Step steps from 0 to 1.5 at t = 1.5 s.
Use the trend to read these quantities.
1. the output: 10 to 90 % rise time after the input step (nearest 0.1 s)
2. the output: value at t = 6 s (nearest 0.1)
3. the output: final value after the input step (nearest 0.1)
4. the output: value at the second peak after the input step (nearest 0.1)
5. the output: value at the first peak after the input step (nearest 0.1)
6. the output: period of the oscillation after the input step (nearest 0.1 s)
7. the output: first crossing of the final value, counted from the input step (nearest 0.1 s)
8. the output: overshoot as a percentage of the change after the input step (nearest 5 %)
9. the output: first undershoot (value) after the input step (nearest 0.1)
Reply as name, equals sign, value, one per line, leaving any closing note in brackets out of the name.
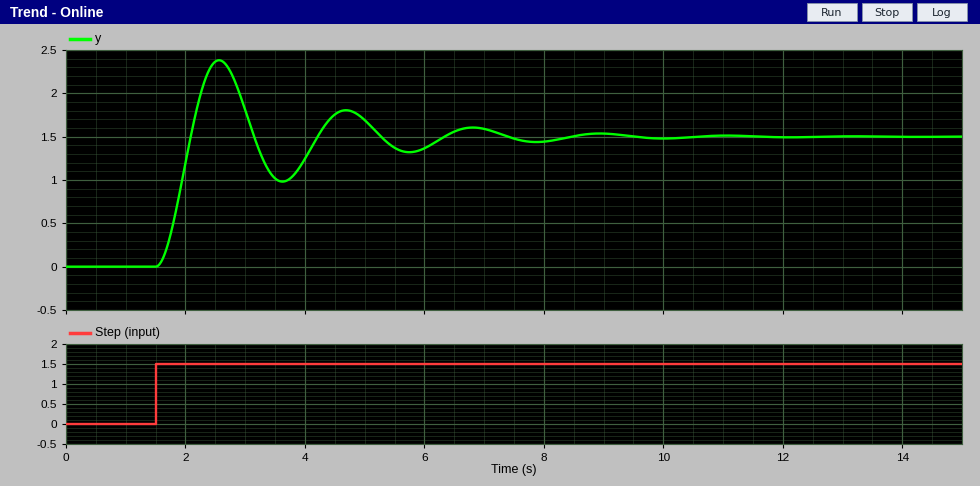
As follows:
the output: 10 to 90 % rise time after the input step = 0.4 s
the output: value at t = 6 s = 1.4
the output: final value after the input step = 1.5
the output: value at the second peak after the input step = 1.8
the output: value at the first peak after the input step = 2.4
the output: period of the oscillation after the input step = 2.1 s
the output: first crossing of the final value, counted from the input step = 0.6 s
the output: overshoot as a percentage of the change after the input step = 60 %
the output: first undershoot (value) after the input step = 1.0
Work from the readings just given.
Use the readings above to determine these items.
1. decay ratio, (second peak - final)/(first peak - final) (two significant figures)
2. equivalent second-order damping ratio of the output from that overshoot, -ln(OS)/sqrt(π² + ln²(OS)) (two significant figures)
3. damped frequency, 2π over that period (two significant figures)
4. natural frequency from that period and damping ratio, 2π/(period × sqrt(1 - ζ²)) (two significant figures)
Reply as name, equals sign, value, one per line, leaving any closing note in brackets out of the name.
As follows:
decay ratio, (second peak - final)/(first peak - final) = 0.33
equivalent second-order damping ratio of the output from that overshoot, -ln(OS)/sqrt(π² + ln²(OS)) = 0.16
damped frequency, 2π over that period = 3.0 rad/s
natural frequency from that period and damping ratio, 2π/(period × sqrt(1 - ζ²)) = 3.0 rad/s
